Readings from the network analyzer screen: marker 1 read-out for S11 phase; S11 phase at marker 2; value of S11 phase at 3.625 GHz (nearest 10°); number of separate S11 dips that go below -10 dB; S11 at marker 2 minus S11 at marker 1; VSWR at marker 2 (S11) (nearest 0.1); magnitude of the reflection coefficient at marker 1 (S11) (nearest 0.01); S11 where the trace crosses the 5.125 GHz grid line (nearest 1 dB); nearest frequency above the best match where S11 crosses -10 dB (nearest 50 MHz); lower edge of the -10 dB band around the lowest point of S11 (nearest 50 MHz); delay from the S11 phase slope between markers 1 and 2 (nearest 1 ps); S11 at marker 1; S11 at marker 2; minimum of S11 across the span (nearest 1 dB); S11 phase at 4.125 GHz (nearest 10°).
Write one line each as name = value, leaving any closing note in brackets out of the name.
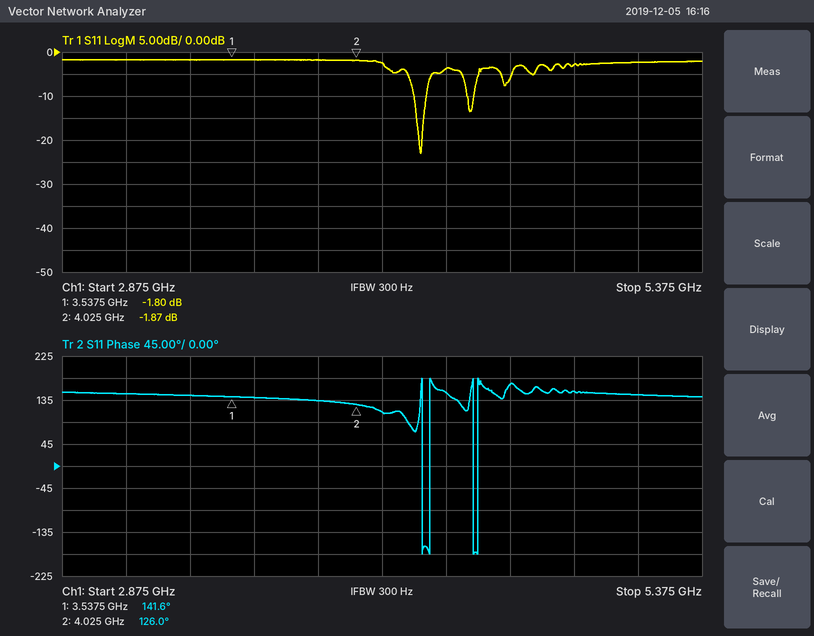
marker 1 read-out for S11 phase = 141.6°
S11 phase at marker 2 = 126.0°
value of S11 phase at 3.625 GHz = 140°
number of separate S11 dips that go below -10 dB = 2
S11 at marker 2 minus S11 at marker 1 = -0.07 dB
VSWR at marker 2 (S11) = 9.3
magnitude of the reflection coefficient at marker 1 (S11) = 0.81
S11 where the trace crosses the 5.125 GHz grid line = -2 dB
nearest frequency above the best match where S11 crosses -10 dB = 4.30 GHz
lower edge of the -10 dB band around the lowest point of S11 = 4.25 GHz
delay from the S11 phase slope between markers 1 and 2 = 89 ps
S11 at marker 1 = -1.80 dB
S11 at marker 2 = -1.87 dB
minimum of S11 across the span = -23 dB
S11 phase at 4.125 GHz = 110°
